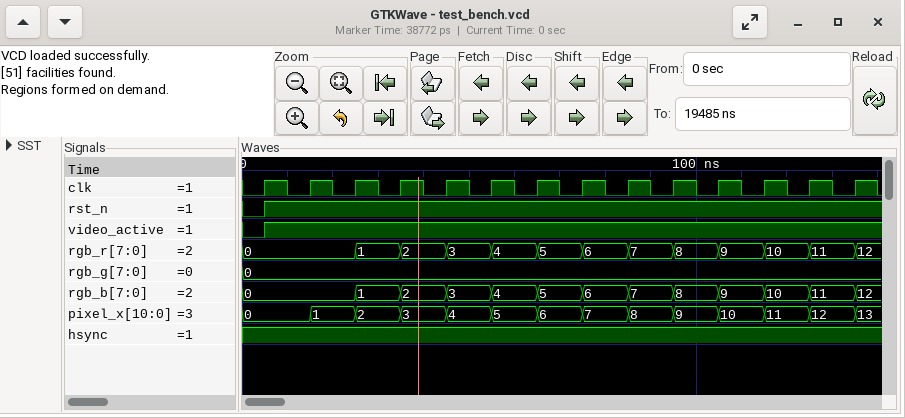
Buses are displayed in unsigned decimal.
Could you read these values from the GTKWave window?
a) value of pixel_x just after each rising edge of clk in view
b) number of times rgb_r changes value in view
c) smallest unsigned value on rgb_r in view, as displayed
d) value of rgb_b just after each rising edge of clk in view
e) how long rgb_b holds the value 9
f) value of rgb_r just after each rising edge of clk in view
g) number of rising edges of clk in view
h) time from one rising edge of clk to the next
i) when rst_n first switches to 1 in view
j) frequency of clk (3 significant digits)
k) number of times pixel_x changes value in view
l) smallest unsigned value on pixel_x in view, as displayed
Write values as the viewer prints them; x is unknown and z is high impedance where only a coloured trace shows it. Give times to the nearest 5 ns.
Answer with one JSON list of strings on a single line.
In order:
["0, 1, 2, 3, 4, 5, 6, 7, 8, 9, 10, 11, 12, 13", "12", "0", "0, 0, 1, 2, 3, 4, 5, 6, 7, 8, 9, 10, 11, 12", "10 ns", "0, 0, 1, 2, 3, 4, 5, 6, 7, 8, 9, 10, 11, 12", "14", "10 ns", "5 ns", "100 MHz", "13", "0"]
